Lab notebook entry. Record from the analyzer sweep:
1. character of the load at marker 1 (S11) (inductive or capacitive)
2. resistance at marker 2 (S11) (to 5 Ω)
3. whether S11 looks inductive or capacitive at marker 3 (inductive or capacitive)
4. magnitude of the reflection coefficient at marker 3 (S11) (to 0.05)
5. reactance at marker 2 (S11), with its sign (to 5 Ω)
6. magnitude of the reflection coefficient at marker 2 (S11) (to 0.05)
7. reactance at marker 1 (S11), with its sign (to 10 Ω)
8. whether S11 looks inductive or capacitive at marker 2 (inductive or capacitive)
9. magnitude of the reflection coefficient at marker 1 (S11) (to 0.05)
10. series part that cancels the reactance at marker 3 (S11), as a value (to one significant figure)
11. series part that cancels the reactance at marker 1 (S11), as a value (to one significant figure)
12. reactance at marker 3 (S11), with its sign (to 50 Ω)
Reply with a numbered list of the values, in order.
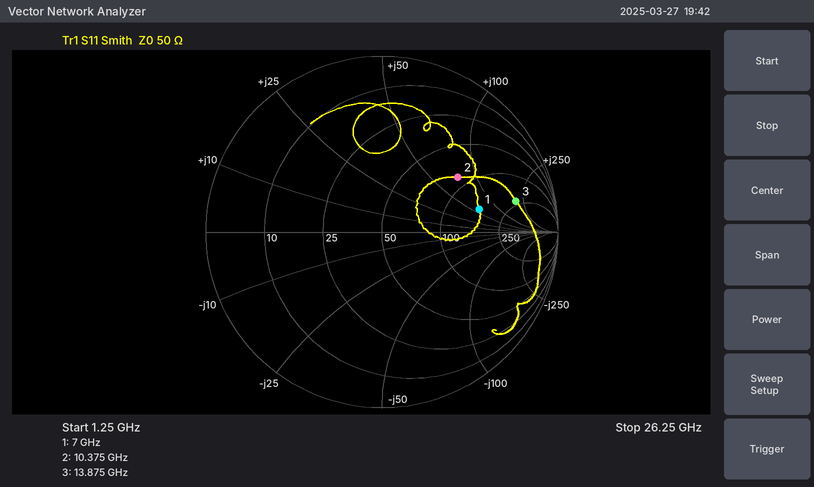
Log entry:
1. inductive
2. 85 Ω
3. inductive
4. 0.80
5. +75 Ω
6. 0.55
7. +60 Ω
8. inductive
9. 0.55
10. 60 fF
11. 400 fF
12. +200 Ω
